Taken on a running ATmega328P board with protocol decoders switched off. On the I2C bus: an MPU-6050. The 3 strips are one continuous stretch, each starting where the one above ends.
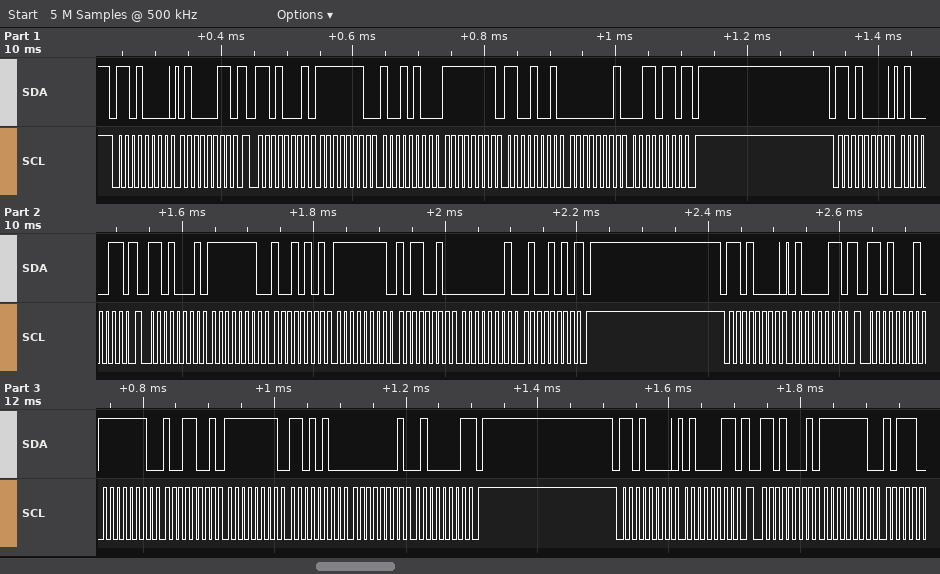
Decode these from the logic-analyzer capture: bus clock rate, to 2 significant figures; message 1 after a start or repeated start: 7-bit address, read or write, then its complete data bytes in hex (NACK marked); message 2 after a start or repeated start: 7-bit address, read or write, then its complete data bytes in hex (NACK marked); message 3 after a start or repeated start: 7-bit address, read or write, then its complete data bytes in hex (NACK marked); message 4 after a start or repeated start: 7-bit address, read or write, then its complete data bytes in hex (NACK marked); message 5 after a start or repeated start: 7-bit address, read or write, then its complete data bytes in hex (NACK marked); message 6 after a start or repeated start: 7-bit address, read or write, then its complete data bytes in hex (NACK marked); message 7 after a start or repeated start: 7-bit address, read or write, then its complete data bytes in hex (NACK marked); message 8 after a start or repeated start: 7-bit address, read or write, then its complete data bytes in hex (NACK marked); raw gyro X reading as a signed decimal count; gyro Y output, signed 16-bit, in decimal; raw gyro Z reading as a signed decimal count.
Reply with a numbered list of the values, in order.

1. 100 kHz
2. 0x68 write: 43
3. 0x68 read: FE 94 FF C9 01 36 NACK
4. 0x68 write: 43
5. 0x68 read: FE 95 FF B2 01 4A NACK
6. 0x68 write: 43
7. 0x68 read: FE 99 FF D4 01 41 NACK
8. 0x68 write: 43
9. 0x68 read: FE
10. -364
11. -55
12. 310
